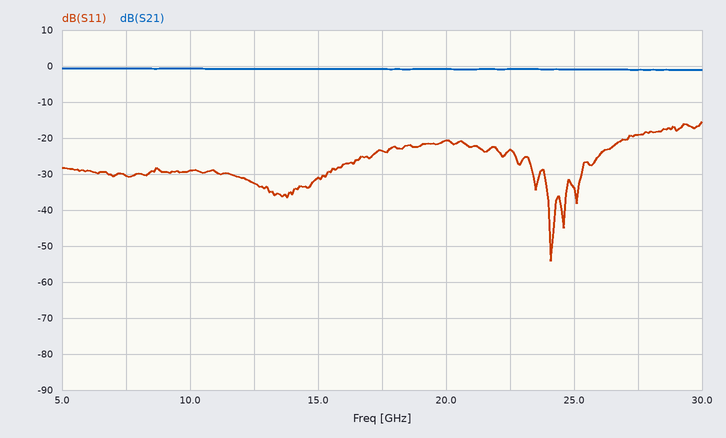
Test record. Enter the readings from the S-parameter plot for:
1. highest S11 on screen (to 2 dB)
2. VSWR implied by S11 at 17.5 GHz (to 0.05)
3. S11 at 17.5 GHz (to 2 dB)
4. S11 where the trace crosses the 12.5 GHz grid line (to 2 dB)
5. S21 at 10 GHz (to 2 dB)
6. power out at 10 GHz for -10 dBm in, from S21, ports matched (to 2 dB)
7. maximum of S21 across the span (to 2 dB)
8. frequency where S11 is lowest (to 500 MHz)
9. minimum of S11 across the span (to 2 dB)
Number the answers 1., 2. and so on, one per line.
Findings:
1. -16 dB
2. 1.15
3. -24 dB
4. -32 dB
5. 0 dB
6. -10 dBm
7. 0 dB
8. 24.0 GHz
9. -54 dB
